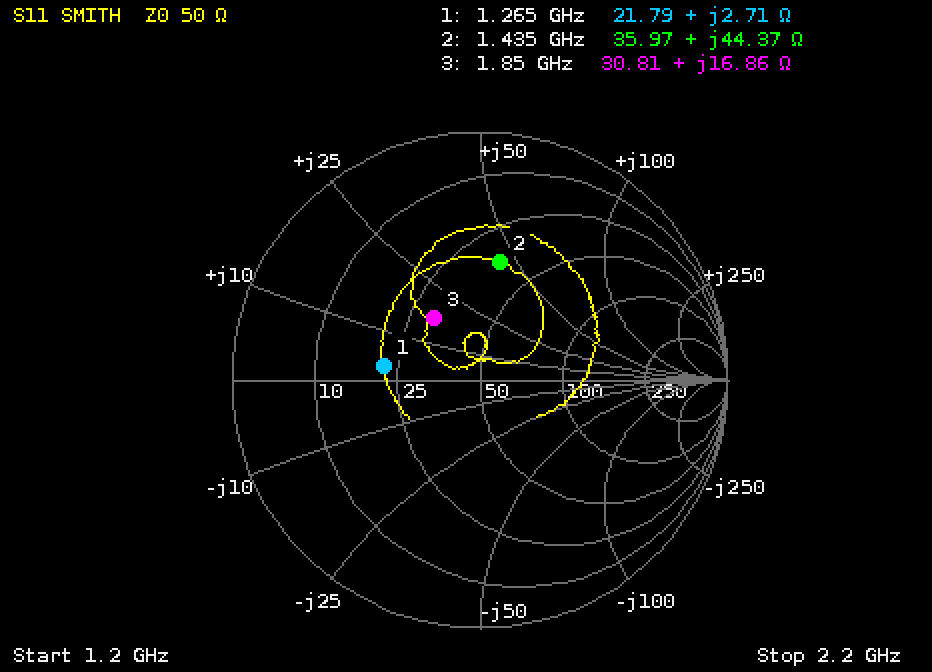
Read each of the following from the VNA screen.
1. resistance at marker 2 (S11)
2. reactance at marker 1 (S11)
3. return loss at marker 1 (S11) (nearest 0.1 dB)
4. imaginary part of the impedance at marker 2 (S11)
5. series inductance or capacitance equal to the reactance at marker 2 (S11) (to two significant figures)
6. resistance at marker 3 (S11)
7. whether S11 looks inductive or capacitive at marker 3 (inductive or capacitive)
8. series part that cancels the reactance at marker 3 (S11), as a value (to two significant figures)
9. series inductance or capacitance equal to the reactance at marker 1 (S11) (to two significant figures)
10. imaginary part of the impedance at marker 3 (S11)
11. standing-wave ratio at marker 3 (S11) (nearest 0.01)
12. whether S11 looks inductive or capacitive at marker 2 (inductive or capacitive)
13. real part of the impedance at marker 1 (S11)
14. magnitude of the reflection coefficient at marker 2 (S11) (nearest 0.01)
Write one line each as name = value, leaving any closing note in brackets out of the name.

resistance at marker 2 = 35.97 Ω
reactance at marker 1 = +2.71 Ω
return loss at marker 1 (S11) = 8.1 dB
imaginary part of the impedance at marker 2 = +44.37 Ω
series inductance or capacitance equal to the reactance at marker 2 (S11) = 4.9 nH
resistance at marker 3 = 30.81 Ω
whether S11 looks inductive or capacitive at marker 3 = inductive
series part that cancels the reactance at marker 3 (S11), as a value = 5.1 pF
series inductance or capacitance equal to the reactance at marker 1 (S11) = 340 pH
imaginary part of the impedance at marker 3 = +16.86 Ω
standing-wave ratio at marker 3 (S11) = 1.90
whether S11 looks inductive or capacitive at marker 2 = inductive
real part of the impedance at marker 1 = 21.79 Ω
magnitude of the reflection coefficient at marker 2 (S11) = 0.48
